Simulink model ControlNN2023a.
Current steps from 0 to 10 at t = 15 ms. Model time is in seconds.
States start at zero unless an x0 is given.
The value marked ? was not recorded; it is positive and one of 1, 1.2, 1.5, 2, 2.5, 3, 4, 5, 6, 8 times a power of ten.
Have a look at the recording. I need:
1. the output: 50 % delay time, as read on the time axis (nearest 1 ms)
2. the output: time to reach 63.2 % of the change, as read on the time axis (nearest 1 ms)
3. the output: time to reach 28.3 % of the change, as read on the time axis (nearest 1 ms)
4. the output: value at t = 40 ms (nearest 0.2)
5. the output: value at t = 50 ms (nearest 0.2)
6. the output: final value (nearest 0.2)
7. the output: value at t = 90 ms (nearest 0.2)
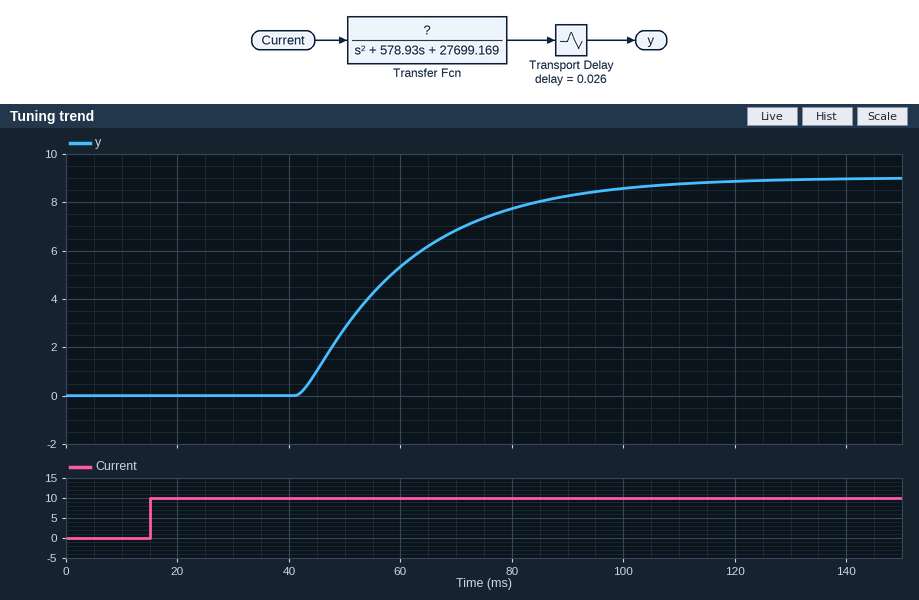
56 ms
62 ms
49 ms
0.0
2.8
9.0
8.2
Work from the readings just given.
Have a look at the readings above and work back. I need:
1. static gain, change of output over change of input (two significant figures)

0.90
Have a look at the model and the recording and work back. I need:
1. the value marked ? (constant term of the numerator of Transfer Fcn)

25000
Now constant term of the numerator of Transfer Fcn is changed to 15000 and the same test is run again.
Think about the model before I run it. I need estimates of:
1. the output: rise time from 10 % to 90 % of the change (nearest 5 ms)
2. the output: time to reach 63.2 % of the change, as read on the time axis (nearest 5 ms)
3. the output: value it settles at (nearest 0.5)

40 ms
60 ms
5.5
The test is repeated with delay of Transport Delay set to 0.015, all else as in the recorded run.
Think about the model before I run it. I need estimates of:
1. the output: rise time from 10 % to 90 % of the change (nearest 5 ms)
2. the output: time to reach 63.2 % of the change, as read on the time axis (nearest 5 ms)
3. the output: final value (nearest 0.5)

40 ms
50 ms
9.0
